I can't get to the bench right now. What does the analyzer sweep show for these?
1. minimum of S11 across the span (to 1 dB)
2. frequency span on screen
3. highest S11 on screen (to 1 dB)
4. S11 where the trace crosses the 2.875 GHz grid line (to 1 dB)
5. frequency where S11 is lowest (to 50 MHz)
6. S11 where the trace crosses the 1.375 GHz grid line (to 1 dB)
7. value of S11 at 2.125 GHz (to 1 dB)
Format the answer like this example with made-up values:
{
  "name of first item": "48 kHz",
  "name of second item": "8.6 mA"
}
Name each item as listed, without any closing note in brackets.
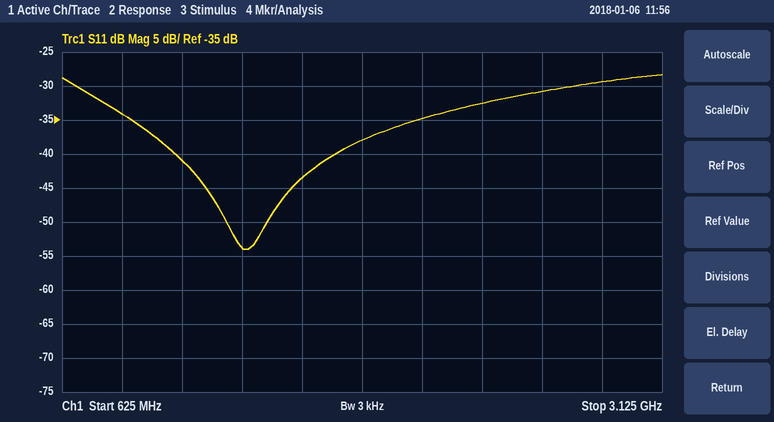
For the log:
{
  "minimum of S11 across the span": "-54 dB",
  "frequency span on screen": "2.5 GHz",
  "highest S11 on screen": "-28 dB",
  "S11 where the trace crosses the 2.875 GHz grid line": "-29 dB",
  "frequency where S11 is lowest": "1.40 GHz",
  "S11 where the trace crosses the 1.375 GHz grid line": "-54 dB",
  "value of S11 at 2.125 GHz": "-35 dB"
}
